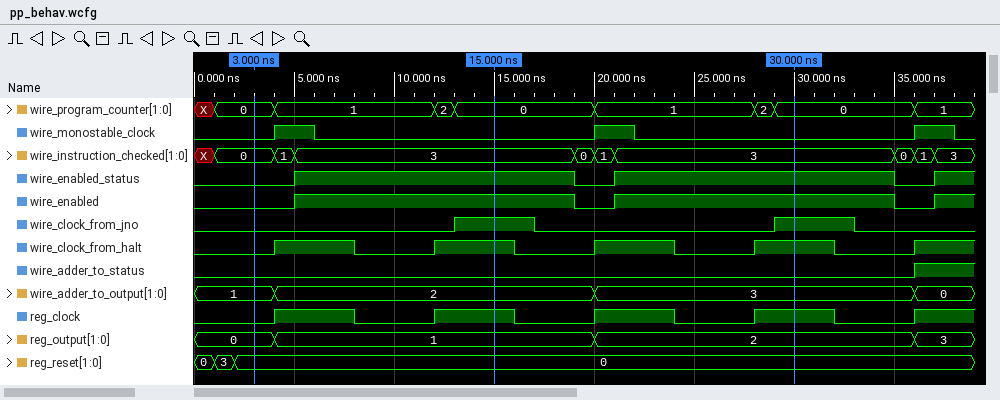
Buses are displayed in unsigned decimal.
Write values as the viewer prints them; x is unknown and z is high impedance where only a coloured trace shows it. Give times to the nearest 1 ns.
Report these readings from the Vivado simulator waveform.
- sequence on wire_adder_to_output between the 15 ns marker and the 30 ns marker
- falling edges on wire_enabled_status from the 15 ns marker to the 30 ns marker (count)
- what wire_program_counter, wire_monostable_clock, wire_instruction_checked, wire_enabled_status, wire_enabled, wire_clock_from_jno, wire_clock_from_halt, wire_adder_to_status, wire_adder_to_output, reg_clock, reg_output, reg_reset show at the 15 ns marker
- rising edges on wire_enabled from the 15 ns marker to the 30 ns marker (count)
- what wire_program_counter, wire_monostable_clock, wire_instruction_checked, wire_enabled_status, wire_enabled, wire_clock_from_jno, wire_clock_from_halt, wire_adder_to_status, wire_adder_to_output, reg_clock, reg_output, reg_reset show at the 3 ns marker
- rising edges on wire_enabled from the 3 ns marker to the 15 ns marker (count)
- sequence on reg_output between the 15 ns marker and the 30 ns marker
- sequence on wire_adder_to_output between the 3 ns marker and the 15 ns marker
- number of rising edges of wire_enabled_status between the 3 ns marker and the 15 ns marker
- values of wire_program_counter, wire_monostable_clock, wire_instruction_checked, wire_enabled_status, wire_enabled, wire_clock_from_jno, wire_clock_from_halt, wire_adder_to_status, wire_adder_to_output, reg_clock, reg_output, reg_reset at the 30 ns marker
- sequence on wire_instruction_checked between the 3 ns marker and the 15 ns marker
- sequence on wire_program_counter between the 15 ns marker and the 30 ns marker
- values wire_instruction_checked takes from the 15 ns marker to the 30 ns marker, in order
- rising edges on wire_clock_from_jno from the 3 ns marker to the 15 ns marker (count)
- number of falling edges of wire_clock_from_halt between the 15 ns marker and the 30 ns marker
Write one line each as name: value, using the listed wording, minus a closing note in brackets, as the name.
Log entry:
sequence on wire_adder_to_output between the 15 ns marker and the 30 ns marker: 2, 3
falling edges on wire_enabled_status from the 15 ns marker to the 30 ns marker: 1
what wire_program_counter, wire_monostable_clock, wire_instruction_checked, wire_enabled_status, wire_enabled, wire_clock_from_jno, wire_clock_from_halt, wire_adder_to_status, wire_adder_to_output, reg_clock, reg_output, reg_reset show at the 15 ns marker: wire_program_counter=0, wire_monostable_clock=0, wire_instruction_checked=3, wire_enabled_status=1, wire_enabled=1, wire_clock_from_jno=1, wire_clock_from_halt=1, wire_adder_to_status=0, wire_adder_to_output=2, reg_clock=1, reg_output=1, reg_reset=0
rising edges on wire_enabled from the 15 ns marker to the 30 ns marker: 1
what wire_program_counter, wire_monostable_clock, wire_instruction_checked, wire_enabled_status, wire_enabled, wire_clock_from_jno, wire_clock_from_halt, wire_adder_to_status, wire_adder_to_output, reg_clock, reg_output, reg_reset show at the 3 ns marker: wire_program_counter=0, wire_monostable_clock=0, wire_instruction_checked=0, wire_enabled_status=0, wire_enabled=0, wire_clock_from_jno=0, wire_clock_from_halt=0, wire_adder_to_status=0, wire_adder_to_output=1, reg_clock=0, reg_output=0, reg_reset=0
rising edges on wire_enabled from the 3 ns marker to the 15 ns marker: 1
sequence on reg_output between the 15 ns marker and the 30 ns marker: 1, 2
sequence on wire_adder_to_output between the 3 ns marker and the 15 ns marker: 1, 2
number of rising edges of wire_enabled_status between the 3 ns marker and the 15 ns marker: 1
values of wire_program_counter, wire_monostable_clock, wire_instruction_checked, wire_enabled_status, wire_enabled, wire_clock_from_jno, wire_clock_from_halt, wire_adder_to_status, wire_adder_to_output, reg_clock, reg_output, reg_reset at the 30 ns marker: wire_program_counter=0, wire_monostable_clock=0, wire_instruction_checked=3, wire_enabled_status=1, wire_enabled=1, wire_clock_from_jno=1, wire_clock_from_halt=1, wire_adder_to_status=0, wire_adder_to_output=3, reg_clock=1, reg_output=2, reg_reset=0
sequence on wire_instruction_checked between the 3 ns marker and the 15 ns marker: 0, 1, 3
sequence on wire_program_counter between the 15 ns marker and the 30 ns marker: 0, 1, 2, 0
values wire_instruction_checked takes from the 15 ns marker to the 30 ns marker, in order: 3, 0, 1, 3
rising edges on wire_clock_from_jno from the 3 ns marker to the 15 ns marker: 1
number of falling edges of wire_clock_from_halt between the 15 ns marker and the 30 ns marker: 2
